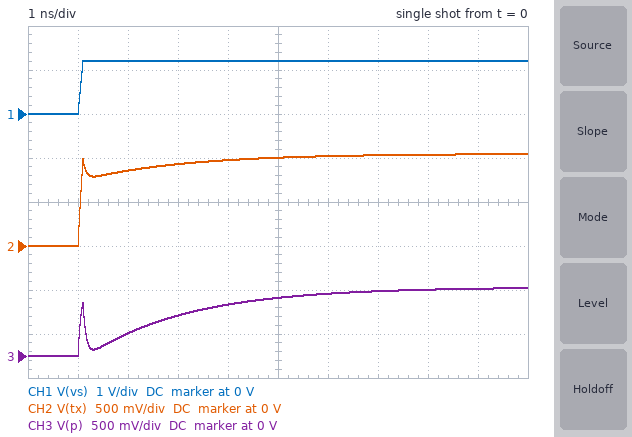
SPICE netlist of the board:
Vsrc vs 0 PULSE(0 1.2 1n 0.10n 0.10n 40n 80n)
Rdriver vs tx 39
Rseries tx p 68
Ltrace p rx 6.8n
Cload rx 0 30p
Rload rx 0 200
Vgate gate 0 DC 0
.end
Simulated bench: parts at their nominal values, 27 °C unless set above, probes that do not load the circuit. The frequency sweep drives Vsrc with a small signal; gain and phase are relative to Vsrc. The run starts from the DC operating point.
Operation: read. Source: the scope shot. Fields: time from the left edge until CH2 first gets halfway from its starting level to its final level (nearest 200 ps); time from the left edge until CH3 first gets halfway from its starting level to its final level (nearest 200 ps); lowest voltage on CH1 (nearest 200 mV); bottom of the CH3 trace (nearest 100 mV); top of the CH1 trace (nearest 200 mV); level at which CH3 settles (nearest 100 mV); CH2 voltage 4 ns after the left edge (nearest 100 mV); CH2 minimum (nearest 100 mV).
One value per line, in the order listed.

1.0 ns
1.0 ns
0 V
0 V
1.2 V
800 mV
1.0 V
0 V
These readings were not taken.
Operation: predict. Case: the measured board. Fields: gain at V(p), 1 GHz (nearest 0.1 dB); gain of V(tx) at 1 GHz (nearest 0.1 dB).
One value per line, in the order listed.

-9.6 dB
-3.3 dB
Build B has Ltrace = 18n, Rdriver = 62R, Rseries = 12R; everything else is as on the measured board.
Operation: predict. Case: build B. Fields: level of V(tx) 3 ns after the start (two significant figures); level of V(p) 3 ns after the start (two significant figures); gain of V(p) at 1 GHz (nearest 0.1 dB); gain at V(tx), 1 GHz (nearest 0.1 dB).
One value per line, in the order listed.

650 mV
550 mV
-1.7 dB
-1.6 dB
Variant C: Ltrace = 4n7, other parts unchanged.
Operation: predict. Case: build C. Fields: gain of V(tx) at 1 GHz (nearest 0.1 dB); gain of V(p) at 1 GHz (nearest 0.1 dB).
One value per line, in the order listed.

-3.6 dB
-13.1 dB
